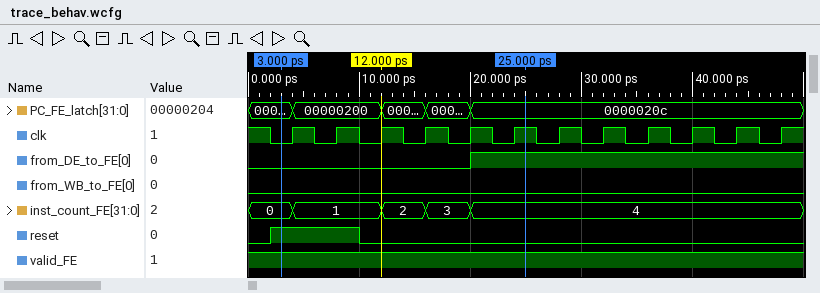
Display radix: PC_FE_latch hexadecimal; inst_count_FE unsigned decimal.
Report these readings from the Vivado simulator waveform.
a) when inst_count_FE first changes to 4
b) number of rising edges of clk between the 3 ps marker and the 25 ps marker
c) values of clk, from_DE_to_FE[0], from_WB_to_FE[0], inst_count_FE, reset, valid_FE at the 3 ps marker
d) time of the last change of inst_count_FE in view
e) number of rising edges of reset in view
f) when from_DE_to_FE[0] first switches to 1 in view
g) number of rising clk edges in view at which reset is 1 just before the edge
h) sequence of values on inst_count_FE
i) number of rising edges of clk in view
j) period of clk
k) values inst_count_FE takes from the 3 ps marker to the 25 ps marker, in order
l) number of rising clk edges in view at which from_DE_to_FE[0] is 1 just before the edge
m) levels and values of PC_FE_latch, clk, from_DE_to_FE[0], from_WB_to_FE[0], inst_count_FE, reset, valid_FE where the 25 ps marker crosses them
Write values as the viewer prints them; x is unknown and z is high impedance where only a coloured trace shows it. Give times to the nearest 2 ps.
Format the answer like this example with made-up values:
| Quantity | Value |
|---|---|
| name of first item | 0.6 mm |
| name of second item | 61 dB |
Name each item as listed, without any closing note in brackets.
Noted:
| Quantity | Value |
|---|---|
| when inst_count_FE first changes to 4 | 20 ps |
| number of rising edges of clk between the 3 ps marker and the 25 ps marker | 6 |
| values of clk, from_DE_to_FE[0], from_WB_to_FE[0], inst_count_FE, reset, valid_FE at the 3 ps marker | clk=0, from_DE_to_FE[0]=0, from_WB_to_FE[0]=0, inst_count_FE=0, reset=1, valid_FE=1 |
| time of the last change of inst_count_FE in view | 20 ps |
| number of rising edges of reset in view | 1 |
| when from_DE_to_FE[0] first switches to 1 in view | 20 ps |
| number of rising clk edges in view at which reset is 1 just before the edge | 2 |
| sequence of values on inst_count_FE | 0, 1, 2, 3, 4 |
| number of rising edges of clk in view | 12 |
| period of clk | 4 ps |
| values inst_count_FE takes from the 3 ps marker to the 25 ps marker, in order | 0, 1, 2, 3, 4 |
| number of rising clk edges in view at which from_DE_to_FE[0] is 1 just before the edge | 7 |
| levels and values of PC_FE_latch, clk, from_DE_to_FE[0], from_WB_to_FE[0], inst_count_FE, reset, valid_FE where the 25 ps marker crosses them | PC_FE_latch=0000020c, clk=1, from_DE_to_FE[0]=1, from_WB_to_FE[0]=0, inst_count_FE=4, reset=0, valid_FE=1 |
